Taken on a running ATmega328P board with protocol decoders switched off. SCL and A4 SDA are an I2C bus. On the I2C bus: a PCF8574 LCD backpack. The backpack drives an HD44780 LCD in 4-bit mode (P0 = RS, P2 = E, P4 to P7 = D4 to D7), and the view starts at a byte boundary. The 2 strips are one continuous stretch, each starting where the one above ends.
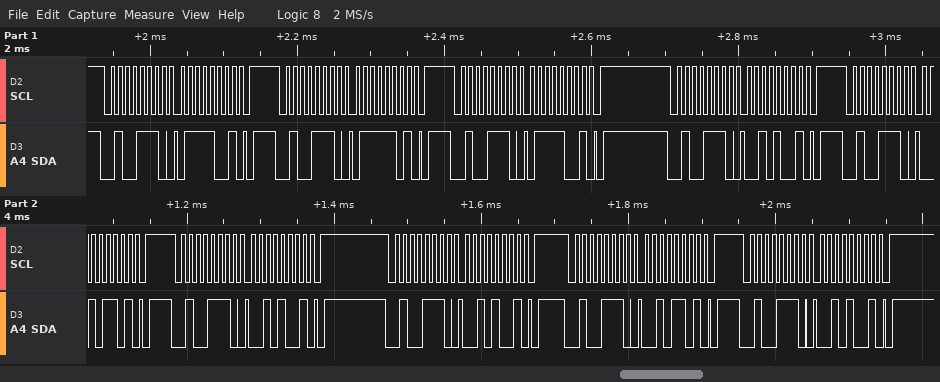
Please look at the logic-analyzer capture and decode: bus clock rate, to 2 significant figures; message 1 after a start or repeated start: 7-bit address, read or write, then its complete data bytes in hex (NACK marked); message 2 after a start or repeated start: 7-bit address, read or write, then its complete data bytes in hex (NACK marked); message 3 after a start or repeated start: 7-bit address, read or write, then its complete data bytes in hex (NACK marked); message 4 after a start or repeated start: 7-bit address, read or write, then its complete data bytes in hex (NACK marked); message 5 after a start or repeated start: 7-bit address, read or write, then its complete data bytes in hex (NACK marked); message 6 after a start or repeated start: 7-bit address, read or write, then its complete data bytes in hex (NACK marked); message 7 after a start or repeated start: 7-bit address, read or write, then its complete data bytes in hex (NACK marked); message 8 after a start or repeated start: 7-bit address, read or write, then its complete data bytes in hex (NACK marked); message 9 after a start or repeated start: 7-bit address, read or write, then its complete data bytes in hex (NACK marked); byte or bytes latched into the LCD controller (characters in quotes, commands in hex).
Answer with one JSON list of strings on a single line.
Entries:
["100 kHz", "0x27 write: 79", "0x27 write: 7D", "0x27 write: 79", "0x27 write: 29", "0x27 write: 2D", "0x27 write: 29", "0x27 write: 29", "0x27 write: 2D", "0x27 write: 29", "'r'"]
